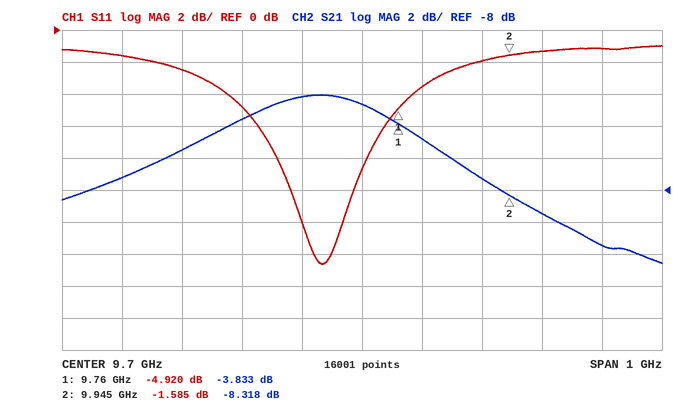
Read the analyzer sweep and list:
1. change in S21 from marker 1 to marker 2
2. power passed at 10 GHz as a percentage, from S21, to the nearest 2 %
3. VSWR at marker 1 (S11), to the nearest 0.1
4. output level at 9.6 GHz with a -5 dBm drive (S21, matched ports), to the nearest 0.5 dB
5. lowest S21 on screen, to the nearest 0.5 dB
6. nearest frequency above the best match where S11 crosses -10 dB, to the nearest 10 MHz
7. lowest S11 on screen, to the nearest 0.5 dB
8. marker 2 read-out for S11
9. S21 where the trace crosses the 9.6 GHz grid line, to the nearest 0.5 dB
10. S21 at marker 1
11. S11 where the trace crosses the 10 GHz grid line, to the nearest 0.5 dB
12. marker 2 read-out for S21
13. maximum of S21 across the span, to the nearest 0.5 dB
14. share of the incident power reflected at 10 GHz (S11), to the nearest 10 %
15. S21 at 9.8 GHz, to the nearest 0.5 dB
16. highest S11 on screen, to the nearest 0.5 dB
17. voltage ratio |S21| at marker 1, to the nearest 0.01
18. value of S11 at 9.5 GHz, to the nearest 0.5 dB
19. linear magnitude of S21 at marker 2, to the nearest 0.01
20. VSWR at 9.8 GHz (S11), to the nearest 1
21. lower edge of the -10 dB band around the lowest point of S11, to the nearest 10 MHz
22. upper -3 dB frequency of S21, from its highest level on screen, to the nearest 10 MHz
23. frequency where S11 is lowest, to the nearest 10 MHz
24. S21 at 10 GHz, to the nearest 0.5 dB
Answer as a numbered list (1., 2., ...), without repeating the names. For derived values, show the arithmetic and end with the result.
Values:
1. -8.318 − (-3.833) = -4.485 dB
2. 10^(-9.5/10) ≈ 11.2 %, so 12 % to the nearest 2 %
3. (1 + 0.5675)/(1 − 0.5675) ≈ 3.6
4. -5 dBm + (-2.0 dB) = -7.0 dBm
5. -12.5 dB
6. 9.69 GHz
7. -14.5 dB
8. -1.585 dB
9. -2.0 dB
10. -3.833 dB
11. -1.5 dB
12. -8.318 dB
13. -2.0 dB
14. 10^(-1.5/10) ≈ 70.8 %, so 70 % to the nearest 10 %
15. -5.0 dB
16. -1.0 dB
17. 10^(-3.833/20) ≈ 0.64
18. -5.0 dB
19. 10^(-8.318/20) ≈ 0.38
20. |Γ| = 10^(-3.5/20) = 0.6683; VSWR = (1 + 0.6683)/(1 − 0.6683) ≈ 5
21. 9.58 GHz
22. 9.81 GHz
23. 9.63 GHz
24. -9.5 dB
